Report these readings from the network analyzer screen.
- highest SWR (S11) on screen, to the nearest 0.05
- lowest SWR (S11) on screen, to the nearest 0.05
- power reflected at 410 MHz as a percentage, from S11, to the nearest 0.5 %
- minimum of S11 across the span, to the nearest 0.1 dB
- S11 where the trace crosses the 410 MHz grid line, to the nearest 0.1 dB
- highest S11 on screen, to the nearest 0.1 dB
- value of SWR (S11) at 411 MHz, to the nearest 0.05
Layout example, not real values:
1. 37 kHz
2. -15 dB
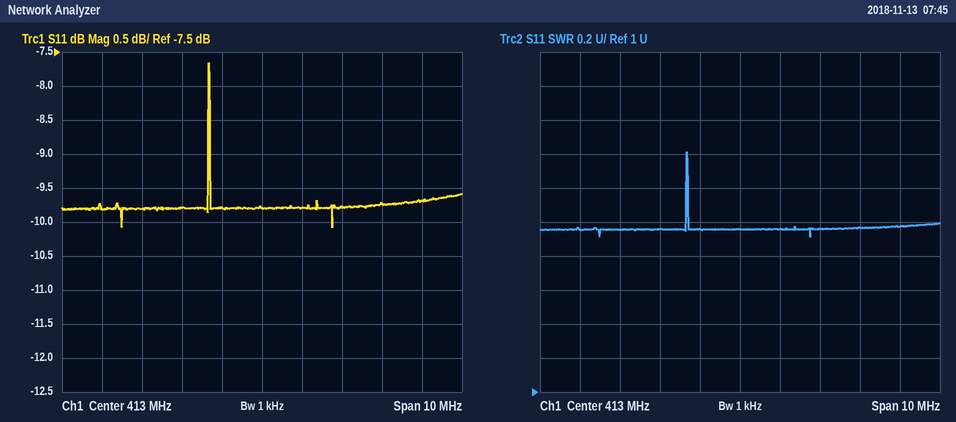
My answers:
1. 2.40
2. 1.90
3. 10.5 %
4. -10.1 dB
5. -9.8 dB
6. -7.7 dB
7. 1.95
